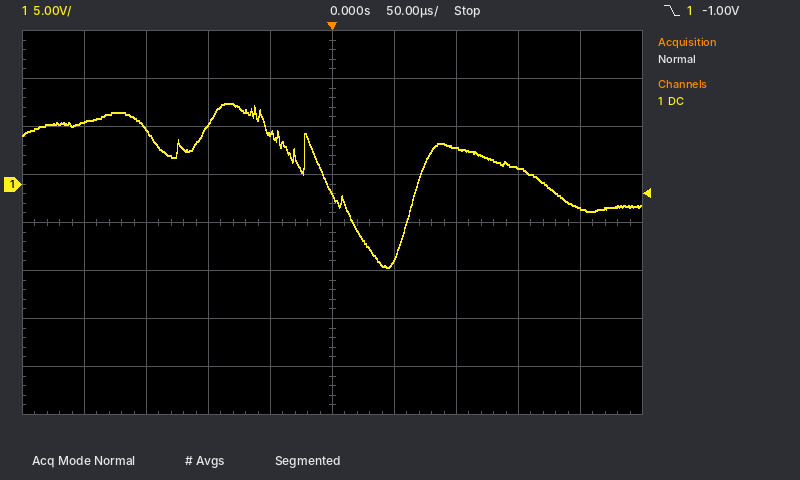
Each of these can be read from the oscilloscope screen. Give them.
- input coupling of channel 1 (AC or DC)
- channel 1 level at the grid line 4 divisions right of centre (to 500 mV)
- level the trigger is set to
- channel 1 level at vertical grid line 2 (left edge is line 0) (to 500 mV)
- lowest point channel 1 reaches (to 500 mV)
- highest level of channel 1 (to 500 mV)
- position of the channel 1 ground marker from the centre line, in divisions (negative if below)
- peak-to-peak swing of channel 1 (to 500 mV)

DC
-2.5 V
-1.00 V
5.5 V
-8.5 V
8.5 V
+0.8 div
17.0 V
